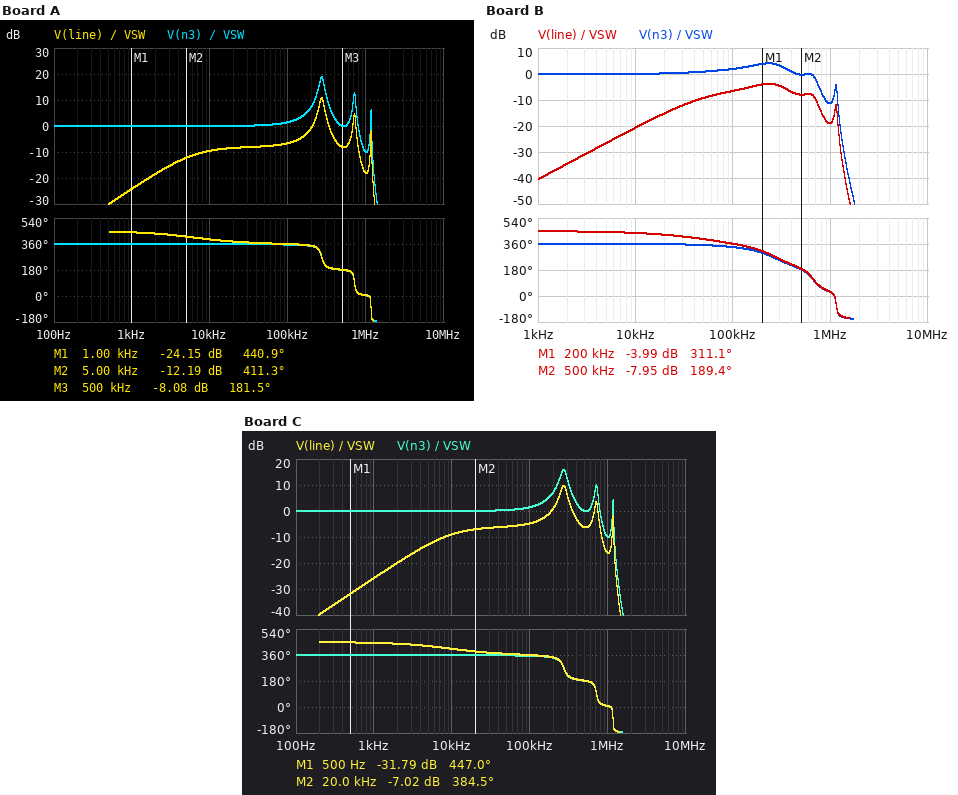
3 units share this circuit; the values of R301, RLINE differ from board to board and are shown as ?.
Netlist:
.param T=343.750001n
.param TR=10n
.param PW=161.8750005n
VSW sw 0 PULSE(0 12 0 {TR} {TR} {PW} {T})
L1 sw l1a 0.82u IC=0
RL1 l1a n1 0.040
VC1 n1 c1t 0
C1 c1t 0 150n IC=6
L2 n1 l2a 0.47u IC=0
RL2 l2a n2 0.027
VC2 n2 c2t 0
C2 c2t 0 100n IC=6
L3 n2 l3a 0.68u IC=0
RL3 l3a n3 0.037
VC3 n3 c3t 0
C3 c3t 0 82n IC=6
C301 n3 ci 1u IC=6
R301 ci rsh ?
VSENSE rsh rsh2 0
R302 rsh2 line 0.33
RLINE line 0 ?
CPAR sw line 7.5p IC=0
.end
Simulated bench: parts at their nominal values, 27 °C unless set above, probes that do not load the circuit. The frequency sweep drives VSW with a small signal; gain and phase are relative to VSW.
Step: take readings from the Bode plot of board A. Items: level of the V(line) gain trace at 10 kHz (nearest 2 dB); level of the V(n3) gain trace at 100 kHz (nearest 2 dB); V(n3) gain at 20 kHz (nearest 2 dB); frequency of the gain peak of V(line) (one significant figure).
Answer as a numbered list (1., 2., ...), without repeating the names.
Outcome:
1. -10 dB
2. 2 dB
3. 0 dB
4. 300 kHz
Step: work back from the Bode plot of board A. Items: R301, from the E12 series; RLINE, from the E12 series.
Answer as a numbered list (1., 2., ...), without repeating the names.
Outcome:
1. 15 Ω
2. 10 Ω
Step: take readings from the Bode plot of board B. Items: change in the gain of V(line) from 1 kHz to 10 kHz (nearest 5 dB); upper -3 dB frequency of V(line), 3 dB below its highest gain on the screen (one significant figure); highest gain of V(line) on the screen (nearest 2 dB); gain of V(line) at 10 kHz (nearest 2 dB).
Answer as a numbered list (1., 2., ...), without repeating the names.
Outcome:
1. 20 dB
2. 400 kHz
3. -4 dB
4. -20 dB
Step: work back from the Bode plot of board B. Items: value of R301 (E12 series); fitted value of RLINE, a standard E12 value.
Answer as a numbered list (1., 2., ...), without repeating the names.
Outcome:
1. 1.8 Ω
2. 1.5 Ω
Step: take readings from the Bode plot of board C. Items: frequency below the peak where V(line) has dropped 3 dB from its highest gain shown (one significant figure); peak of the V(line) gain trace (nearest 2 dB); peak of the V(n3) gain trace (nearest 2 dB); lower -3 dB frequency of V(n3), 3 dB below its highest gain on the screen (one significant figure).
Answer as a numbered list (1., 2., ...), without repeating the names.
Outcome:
1. 200 kHz
2. 10 dB
3. 16 dB
4. 200 kHz
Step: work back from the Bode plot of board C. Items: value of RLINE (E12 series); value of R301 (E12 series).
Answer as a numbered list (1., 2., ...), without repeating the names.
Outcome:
1. 8.2 Ω
2. 8.2 Ω
